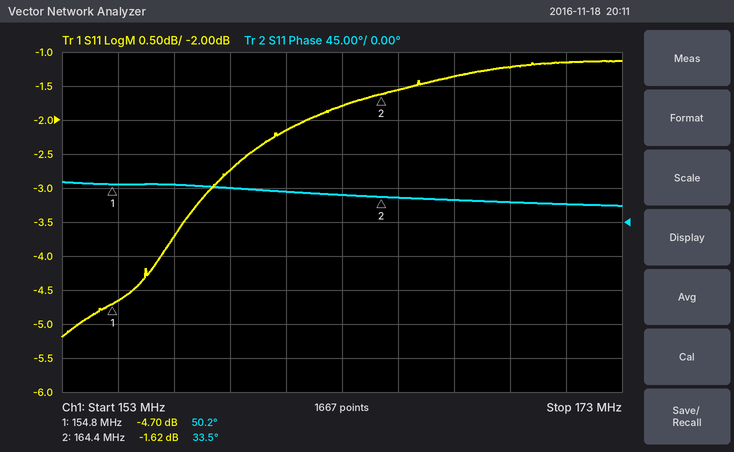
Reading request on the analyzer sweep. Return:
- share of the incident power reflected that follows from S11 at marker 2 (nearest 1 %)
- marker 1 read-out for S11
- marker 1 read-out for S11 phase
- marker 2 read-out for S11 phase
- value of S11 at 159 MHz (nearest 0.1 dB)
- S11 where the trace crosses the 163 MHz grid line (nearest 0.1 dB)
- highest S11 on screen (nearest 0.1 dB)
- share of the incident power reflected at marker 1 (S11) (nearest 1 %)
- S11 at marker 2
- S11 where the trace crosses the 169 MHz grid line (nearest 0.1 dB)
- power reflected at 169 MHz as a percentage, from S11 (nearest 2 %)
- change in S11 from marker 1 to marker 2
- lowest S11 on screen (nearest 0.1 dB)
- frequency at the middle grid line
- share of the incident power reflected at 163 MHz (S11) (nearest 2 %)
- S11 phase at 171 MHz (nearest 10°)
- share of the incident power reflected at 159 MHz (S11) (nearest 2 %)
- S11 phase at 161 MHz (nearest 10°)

69 %
-4.70 dB
50.2°
33.5°
-2.7 dB
-1.8 dB
-1.1 dB
34 %
-1.62 dB
-1.2 dB
76 %
3.08 dB
-5.2 dB
163 MHz
66 %
20°
54 %
40°
